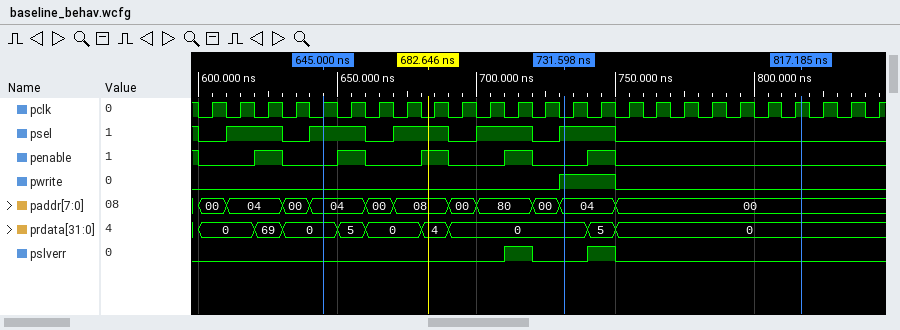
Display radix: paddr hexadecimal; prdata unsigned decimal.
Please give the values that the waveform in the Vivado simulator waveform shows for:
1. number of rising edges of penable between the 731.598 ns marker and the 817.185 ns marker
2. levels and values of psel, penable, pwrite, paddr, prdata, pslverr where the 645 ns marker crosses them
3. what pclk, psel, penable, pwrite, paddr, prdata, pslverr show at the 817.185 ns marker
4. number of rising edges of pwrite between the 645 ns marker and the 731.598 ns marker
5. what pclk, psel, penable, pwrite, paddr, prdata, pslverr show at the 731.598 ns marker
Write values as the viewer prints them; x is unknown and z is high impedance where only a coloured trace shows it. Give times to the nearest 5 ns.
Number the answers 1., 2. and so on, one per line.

1. 1
2. psel=1, penable=0, pwrite=0, paddr=04, prdata=0, pslverr=0
3. pclk=1, psel=0, penable=0, pwrite=0, paddr=00, prdata=0, pslverr=0
4. 1
5. pclk=0, psel=1, penable=0, pwrite=1, paddr=04, prdata=0, pslverr=0
